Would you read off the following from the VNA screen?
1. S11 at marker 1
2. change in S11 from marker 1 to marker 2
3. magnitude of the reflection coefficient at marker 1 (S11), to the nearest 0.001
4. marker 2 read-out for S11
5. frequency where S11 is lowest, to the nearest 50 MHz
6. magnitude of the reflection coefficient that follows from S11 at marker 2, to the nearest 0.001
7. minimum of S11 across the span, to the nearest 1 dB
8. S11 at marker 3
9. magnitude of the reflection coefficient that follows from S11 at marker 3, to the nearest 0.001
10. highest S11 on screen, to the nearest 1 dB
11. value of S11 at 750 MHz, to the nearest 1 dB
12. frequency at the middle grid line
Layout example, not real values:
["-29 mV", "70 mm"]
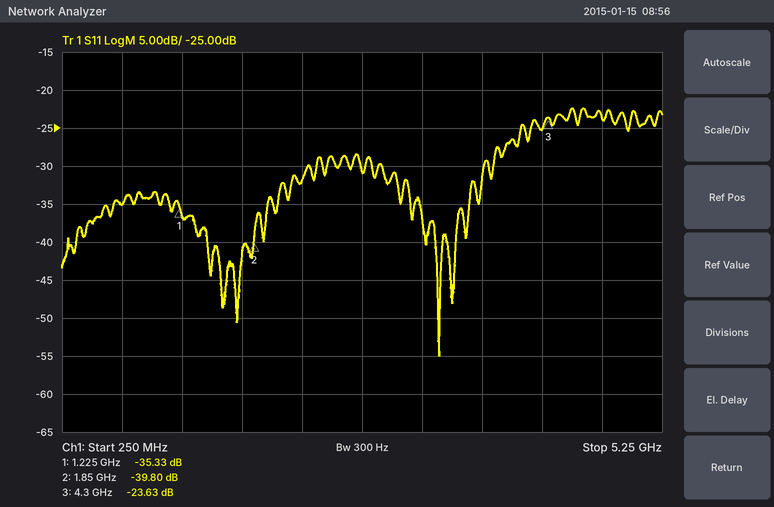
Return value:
["-35.33 dB", "-4.47 dB", "0.017", "-39.80 dB", "3.40 GHz", "0.010", "-55 dB", "-23.63 dB", "0.066", "-22 dB", "-35 dB", "2.75 GHz"]
